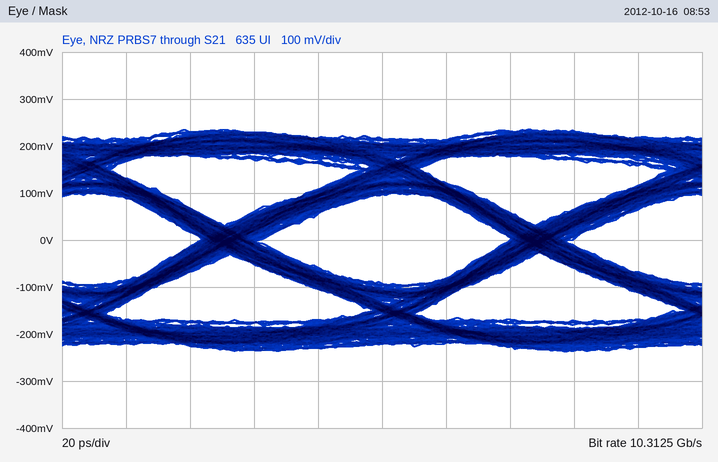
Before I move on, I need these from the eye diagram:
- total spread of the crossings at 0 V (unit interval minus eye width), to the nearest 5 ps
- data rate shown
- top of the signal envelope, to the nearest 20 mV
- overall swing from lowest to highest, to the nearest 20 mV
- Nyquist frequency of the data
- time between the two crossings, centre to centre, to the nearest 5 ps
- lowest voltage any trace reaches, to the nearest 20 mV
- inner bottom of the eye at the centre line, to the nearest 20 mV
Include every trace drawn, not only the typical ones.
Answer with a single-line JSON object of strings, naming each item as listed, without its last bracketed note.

{"total spread of the crossings at 0 V (unit interval minus eye width), to the nearest 5 ps": "20 ps", "data rate shown": "10.3125 Gb/s", "top of the signal envelope, to the nearest 20 mV": "240 mV", "overall swing from lowest to highest, to the nearest 20 mV": "480 mV", "Nyquist frequency of the data": "5.15625 GHz", "time between the two crossings, centre to centre, to the nearest 5 ps": "95 ps", "lowest voltage any trace reaches, to the nearest 20 mV": "-240 mV", "inner bottom of the eye at the centre line, to the nearest 20 mV": "-100 mV"}
